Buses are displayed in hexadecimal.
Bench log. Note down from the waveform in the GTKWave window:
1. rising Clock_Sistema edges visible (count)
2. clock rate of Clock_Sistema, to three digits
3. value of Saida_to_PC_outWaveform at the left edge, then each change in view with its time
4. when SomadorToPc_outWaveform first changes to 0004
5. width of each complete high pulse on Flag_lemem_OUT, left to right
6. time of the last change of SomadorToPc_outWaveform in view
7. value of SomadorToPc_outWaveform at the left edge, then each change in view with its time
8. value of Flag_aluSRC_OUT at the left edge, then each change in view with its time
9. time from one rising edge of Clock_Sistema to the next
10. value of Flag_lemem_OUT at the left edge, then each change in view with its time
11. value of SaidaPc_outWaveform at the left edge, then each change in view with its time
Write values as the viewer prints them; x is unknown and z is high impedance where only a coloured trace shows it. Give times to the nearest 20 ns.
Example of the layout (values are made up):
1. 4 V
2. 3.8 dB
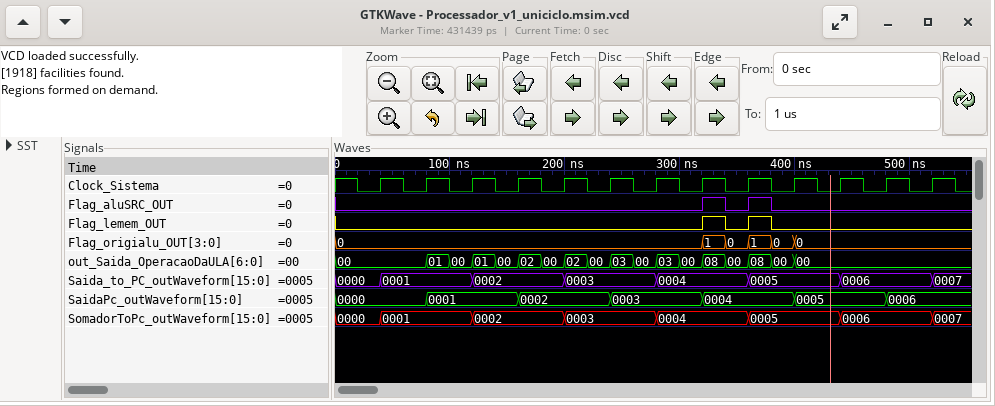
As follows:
1. 13
2. 25.0 MHz
3. 0000, 0001 at 40 ns, 0002 at 120 ns, 0003 at 200 ns, 0004 at 280 ns, 0005 at 360 ns, 0006 at 440 ns, 0007 at 520 ns
4. 280 ns
5. 20 ns, 20 ns
6. 520 ns
7. 0000, 0001 at 40 ns, 0002 at 120 ns, 0003 at 200 ns, 0004 at 280 ns, 0005 at 360 ns, 0006 at 440 ns, 0007 at 520 ns
8. 0, 1 at 320 ns, 0 at 340 ns, 1 at 360 ns, 0 at 380 ns
9. 40 ns
10. 0, 1 at 320 ns, 0 at 340 ns, 1 at 360 ns, 0 at 380 ns
11. 0000, 0001 at 80 ns, 0002 at 160 ns, 0003 at 240 ns, 0004 at 320 ns, 0005 at 400 ns, 0006 at 480 ns
